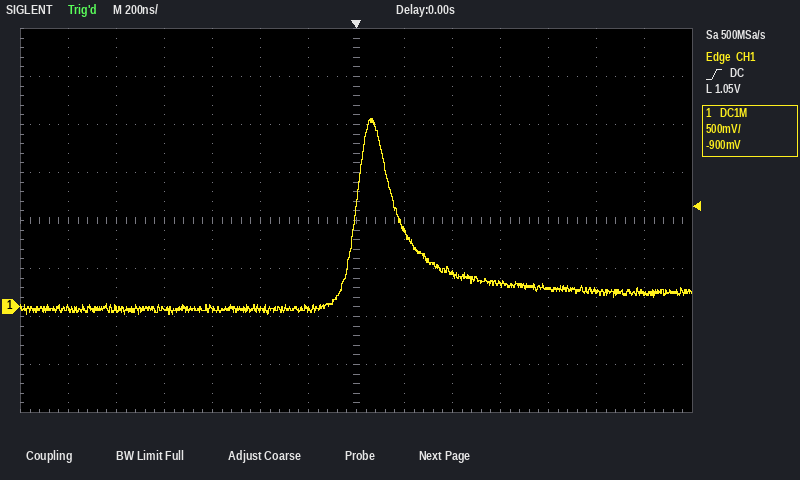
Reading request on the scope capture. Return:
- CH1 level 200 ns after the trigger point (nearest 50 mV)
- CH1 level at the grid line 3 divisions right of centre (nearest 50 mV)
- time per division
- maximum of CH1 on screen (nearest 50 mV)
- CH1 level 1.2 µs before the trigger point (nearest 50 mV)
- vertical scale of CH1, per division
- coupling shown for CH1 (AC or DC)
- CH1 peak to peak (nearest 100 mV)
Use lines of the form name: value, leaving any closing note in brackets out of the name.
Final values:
CH1 level 200 ns after the trigger point: 800 mV
CH1 level at the grid line 3 divisions right of centre: 250 mV
time per division: 200 ns
maximum of CH1 on screen: 1.95 V
CH1 level 1.2 µs before the trigger point: 0 mV
vertical scale of CH1, per division: 500 mV
coupling shown for CH1: DC
CH1 peak to peak: 2.00 V
